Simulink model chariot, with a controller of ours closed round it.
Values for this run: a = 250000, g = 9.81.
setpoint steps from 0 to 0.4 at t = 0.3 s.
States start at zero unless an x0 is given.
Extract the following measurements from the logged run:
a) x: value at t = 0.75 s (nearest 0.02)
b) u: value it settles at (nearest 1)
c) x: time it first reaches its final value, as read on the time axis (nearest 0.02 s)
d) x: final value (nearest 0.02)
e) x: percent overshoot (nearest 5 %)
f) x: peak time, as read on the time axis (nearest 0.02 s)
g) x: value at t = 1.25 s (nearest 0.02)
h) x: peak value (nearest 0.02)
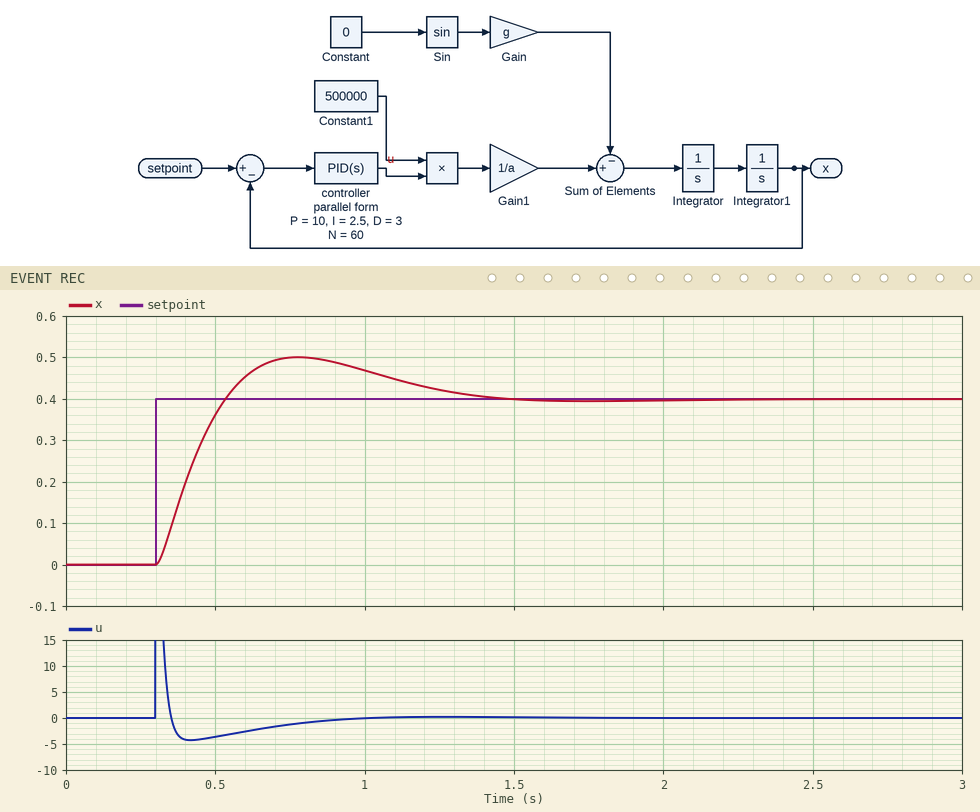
0.50
0
0.54 s
0.40
25 %
0.78 s
0.42
0.50
